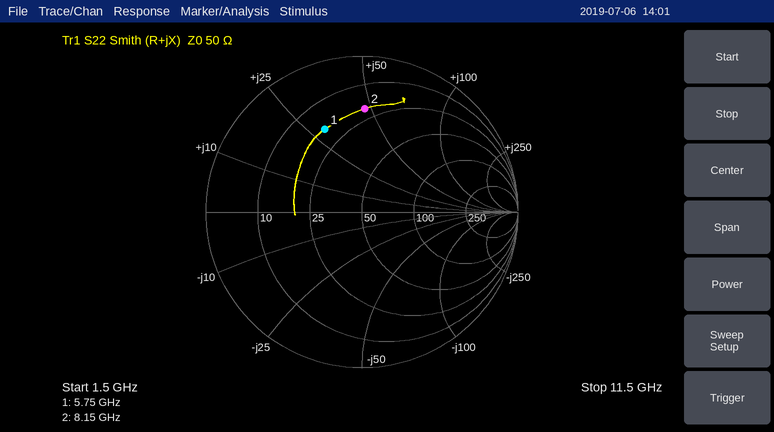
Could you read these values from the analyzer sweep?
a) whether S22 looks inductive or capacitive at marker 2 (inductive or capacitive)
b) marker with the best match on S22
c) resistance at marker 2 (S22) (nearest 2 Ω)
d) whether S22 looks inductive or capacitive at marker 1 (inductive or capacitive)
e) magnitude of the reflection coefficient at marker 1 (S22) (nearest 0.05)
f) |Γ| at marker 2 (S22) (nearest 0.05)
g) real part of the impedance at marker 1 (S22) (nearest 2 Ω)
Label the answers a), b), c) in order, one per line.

a) inductive
b) marker 1
c) 20 Ω
d) inductive
e) 0.60
f) 0.65
g) 18 Ω
